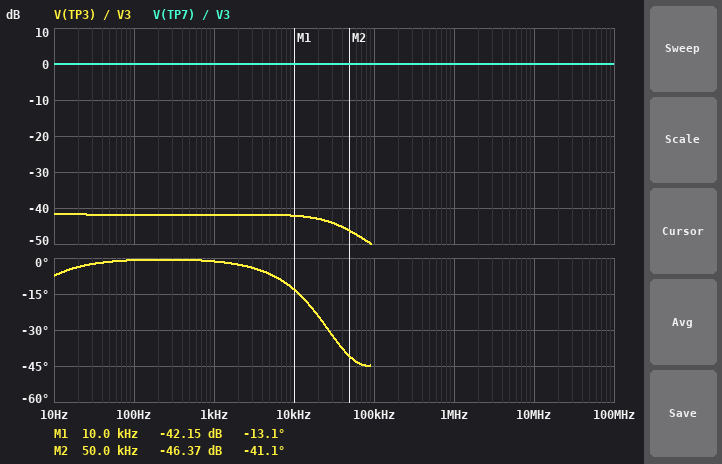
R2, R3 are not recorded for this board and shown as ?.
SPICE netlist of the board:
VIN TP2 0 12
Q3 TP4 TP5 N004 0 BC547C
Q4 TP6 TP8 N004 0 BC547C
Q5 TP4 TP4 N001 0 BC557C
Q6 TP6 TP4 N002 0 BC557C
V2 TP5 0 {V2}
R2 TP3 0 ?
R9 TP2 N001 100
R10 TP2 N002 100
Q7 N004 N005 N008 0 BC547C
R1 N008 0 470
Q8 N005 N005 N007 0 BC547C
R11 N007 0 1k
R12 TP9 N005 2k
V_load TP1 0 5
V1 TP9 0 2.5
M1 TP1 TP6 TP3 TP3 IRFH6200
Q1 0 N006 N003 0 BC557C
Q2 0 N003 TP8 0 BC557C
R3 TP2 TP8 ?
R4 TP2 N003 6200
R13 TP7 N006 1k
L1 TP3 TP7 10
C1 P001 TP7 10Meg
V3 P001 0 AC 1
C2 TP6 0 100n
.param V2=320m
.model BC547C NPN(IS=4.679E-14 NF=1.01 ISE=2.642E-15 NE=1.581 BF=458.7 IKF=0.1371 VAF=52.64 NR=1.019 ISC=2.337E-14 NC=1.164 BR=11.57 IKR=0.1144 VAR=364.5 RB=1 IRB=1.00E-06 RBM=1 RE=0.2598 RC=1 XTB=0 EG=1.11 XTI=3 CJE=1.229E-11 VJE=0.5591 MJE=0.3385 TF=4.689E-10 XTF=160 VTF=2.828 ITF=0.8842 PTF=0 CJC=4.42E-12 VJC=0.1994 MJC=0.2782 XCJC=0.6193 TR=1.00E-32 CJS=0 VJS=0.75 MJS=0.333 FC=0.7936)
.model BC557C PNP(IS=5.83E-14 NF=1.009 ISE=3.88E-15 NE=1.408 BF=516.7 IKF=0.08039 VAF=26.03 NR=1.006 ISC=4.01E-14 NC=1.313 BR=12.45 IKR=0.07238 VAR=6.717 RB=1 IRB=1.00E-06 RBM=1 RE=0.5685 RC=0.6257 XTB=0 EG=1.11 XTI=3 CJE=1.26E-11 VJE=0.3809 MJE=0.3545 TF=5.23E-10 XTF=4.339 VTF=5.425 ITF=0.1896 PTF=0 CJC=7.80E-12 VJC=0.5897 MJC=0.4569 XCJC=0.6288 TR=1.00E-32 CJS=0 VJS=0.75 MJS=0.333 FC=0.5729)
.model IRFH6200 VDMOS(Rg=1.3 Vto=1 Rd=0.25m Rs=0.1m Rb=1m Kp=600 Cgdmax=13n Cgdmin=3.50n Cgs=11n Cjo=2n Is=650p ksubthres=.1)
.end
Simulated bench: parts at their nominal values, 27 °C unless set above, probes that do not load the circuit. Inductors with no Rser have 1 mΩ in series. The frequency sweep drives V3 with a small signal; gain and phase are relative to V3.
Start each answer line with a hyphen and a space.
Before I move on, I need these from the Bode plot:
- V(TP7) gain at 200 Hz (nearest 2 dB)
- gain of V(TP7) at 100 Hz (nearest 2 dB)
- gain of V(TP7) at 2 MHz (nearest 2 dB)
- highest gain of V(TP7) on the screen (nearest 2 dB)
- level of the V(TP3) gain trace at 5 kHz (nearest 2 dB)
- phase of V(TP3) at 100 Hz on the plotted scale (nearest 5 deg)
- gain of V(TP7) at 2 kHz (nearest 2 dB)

- 0 dB
- 0 dB
- 0 dB
- 0 dB
- -42 dB
- 0 deg
- 0 dB
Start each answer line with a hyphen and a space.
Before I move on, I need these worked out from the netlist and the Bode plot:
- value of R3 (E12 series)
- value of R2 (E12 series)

- 3.9 kΩ
- 0.68 Ω
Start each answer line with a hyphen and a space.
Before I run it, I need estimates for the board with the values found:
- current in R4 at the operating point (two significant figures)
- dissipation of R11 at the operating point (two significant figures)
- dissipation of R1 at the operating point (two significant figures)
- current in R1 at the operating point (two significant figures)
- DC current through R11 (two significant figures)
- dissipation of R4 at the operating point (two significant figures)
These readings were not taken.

- 1.8 mA
- 340 µW
- 660 µW
- 1.2 mA
- 590 µA
- 21 mW
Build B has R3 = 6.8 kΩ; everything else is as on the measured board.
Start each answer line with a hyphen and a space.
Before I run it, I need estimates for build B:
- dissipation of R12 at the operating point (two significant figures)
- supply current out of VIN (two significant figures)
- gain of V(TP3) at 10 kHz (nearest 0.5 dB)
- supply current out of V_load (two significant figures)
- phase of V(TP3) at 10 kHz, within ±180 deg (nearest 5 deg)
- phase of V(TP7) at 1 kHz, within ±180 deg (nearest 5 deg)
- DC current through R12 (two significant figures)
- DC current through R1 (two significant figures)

- 880 µW
- 3.4 mA
- -48.5 dB
- 380 µA
- -20 deg
- 0 deg
- 660 µA
- 1.1 mA
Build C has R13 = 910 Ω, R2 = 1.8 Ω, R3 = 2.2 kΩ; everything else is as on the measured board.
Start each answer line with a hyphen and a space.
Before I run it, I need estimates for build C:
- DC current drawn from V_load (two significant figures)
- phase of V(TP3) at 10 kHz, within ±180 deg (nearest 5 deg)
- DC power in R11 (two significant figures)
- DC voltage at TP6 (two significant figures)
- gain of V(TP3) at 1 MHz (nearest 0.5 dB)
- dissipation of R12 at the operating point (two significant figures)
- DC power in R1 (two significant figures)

- 1.0 mA
- -10 deg
- 360 µW
- 600 mV
- -46.0 dB
- 840 µW
- 700 µW
